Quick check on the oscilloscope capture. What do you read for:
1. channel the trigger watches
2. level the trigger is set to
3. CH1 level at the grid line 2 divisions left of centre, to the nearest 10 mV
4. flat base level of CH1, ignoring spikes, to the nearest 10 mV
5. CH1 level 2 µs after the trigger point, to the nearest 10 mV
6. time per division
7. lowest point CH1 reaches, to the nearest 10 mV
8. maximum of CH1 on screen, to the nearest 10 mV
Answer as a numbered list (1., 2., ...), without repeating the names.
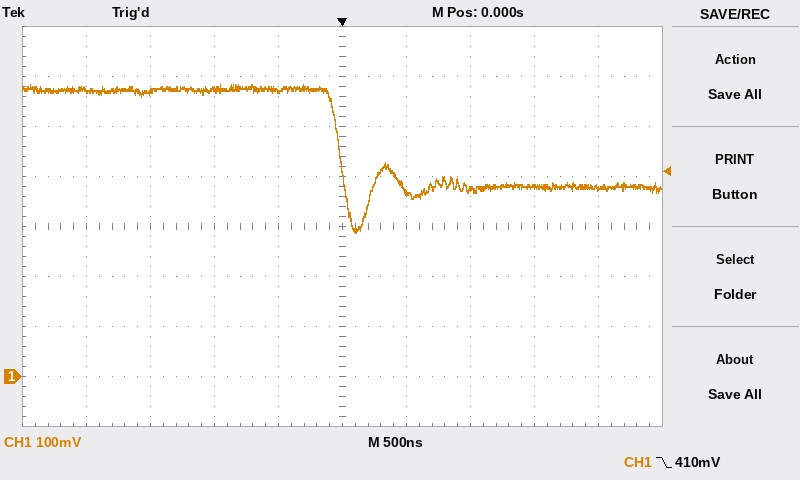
1. CH1
2. 410 mV
3. 570 mV
4. 380 mV
5. 380 mV
6. 500 ns
7. 290 mV
8. 580 mV
